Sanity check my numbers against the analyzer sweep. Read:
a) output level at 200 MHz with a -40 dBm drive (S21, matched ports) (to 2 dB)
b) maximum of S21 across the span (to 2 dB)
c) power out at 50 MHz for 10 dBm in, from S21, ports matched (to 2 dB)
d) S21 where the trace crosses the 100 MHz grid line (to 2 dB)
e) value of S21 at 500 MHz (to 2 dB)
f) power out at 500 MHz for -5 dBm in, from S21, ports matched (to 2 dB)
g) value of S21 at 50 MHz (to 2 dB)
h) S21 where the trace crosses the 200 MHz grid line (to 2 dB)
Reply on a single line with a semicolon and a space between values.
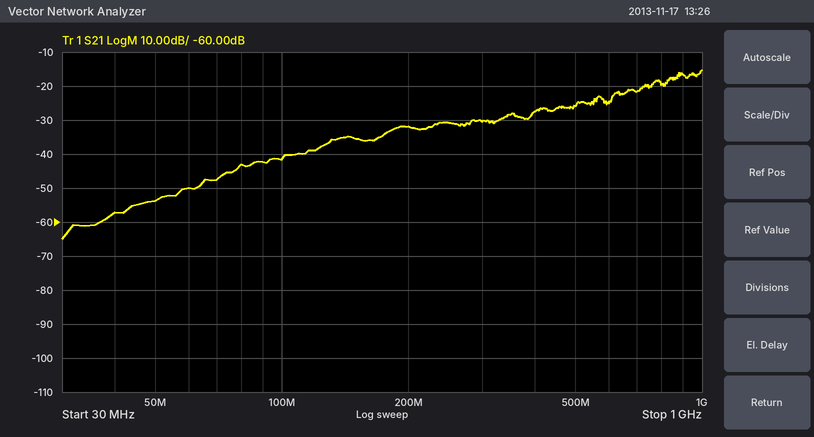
-72 dBm; -16 dB; -44 dBm; -42 dB; -26 dB; -30 dBm; -54 dB; -32 dB
